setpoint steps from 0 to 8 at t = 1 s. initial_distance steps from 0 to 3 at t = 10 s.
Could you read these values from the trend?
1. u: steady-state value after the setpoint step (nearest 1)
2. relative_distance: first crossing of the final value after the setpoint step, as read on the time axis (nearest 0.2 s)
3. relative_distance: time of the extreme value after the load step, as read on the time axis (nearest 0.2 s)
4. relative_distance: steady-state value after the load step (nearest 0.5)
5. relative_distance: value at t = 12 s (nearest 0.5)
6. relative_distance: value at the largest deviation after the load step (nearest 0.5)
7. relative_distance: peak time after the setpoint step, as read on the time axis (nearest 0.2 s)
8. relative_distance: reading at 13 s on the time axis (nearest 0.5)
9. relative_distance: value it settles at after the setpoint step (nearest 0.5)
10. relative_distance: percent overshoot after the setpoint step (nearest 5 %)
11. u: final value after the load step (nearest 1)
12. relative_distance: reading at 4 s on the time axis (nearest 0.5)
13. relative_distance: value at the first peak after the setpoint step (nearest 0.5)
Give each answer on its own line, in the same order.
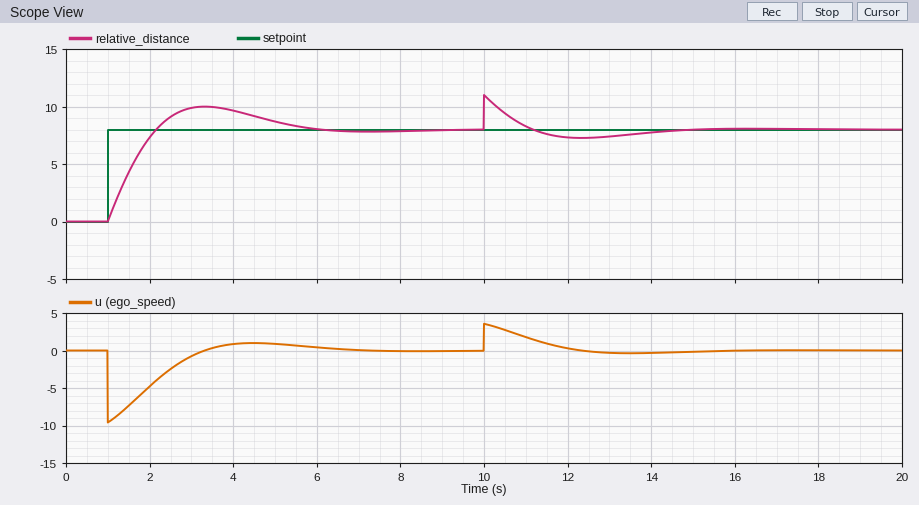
0
2.2 s
10.0 s
8.0
7.5
11.0
3.4 s
7.5
8.0
25 %
0
9.5
10.0
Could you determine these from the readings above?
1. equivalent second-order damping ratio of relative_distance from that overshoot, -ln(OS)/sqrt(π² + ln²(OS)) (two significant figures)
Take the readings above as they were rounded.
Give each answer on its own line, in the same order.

0.40
